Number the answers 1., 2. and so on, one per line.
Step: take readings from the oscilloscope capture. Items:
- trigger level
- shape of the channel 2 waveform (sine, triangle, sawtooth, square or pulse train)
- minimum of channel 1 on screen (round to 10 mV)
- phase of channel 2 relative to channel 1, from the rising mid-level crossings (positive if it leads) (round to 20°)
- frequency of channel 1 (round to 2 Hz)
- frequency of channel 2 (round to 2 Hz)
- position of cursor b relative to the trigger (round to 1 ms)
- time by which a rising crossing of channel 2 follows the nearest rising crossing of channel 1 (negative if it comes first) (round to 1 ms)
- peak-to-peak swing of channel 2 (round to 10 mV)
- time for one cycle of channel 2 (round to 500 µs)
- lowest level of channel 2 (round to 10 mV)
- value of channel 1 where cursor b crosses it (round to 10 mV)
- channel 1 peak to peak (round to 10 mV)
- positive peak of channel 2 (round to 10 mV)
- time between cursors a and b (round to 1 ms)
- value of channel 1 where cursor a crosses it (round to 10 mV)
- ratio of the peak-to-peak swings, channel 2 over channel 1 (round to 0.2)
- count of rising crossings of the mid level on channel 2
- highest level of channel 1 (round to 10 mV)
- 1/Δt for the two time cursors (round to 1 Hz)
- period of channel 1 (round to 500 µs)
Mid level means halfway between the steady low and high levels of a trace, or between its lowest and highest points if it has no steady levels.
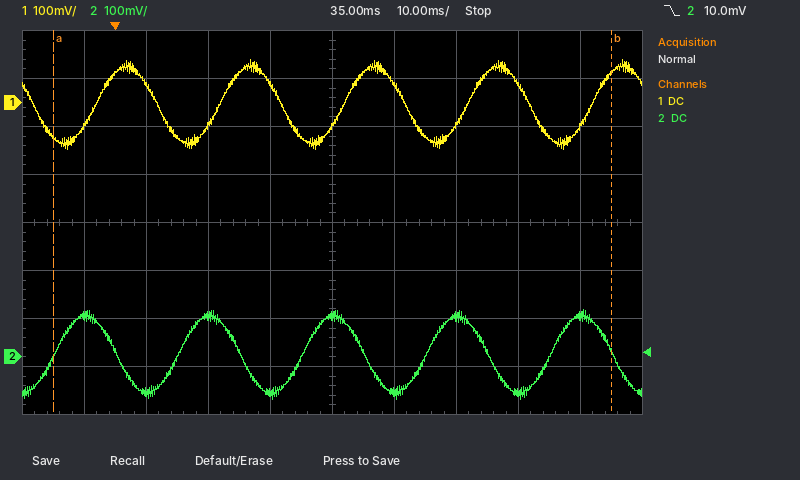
1. 10.0 mV
2. sine
3. -100 mV
4. +120°
5. 50 Hz
6. 50 Hz
7. +80 ms
8. -7 ms
9. 190 mV
10. 20.0 ms
11. -90 mV
12. 60 mV
13. 190 mV
14. 100 mV
15. 90 ms
16. -70 mV
17. 1.0
18. 5
19. 90 mV
20. 11 Hz
21. 20.0 ms
